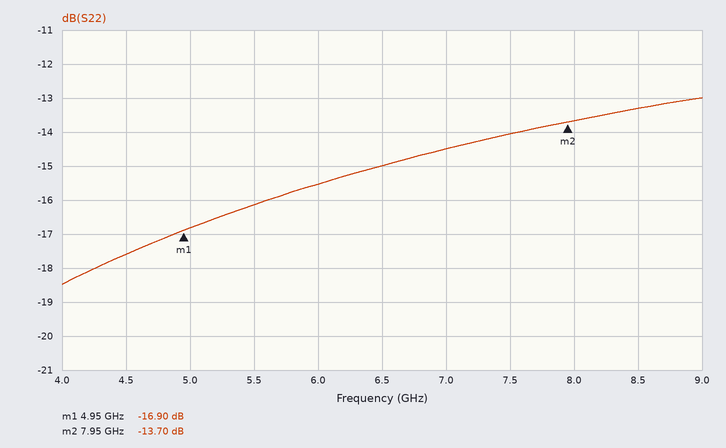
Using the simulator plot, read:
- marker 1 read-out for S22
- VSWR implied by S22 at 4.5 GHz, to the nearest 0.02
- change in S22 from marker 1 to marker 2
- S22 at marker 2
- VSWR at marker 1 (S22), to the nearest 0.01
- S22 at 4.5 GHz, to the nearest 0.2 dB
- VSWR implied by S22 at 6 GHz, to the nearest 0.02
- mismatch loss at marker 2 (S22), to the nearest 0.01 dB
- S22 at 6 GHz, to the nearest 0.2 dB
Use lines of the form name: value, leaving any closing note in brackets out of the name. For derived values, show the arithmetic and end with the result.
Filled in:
marker 1 read-out for S22: -16.90 dB
VSWR implied by S22 at 4.5 GHz, to the nearest 0.02: |Γ| = 10^(-17.6/20) = 0.1318; VSWR = (1 + 0.1318)/(1 − 0.1318) ≈ 1.30
change in S22 from marker 1 to marker 2: -13.7 − (-16.9) = 3.20 dB
S22 at marker 2: -13.70 dB
VSWR at marker 1 (S22), to the nearest 0.01: (1 + 0.1429)/(1 − 0.1429) ≈ 1.33
S22 at 4.5 GHz, to the nearest 0.2 dB: -17.6 dB
VSWR implied by S22 at 6 GHz, to the nearest 0.02: |Γ| = 10^(-15.6/20) = 0.1660; VSWR = (1 + 0.1660)/(1 − 0.1660) ≈ 1.40
mismatch loss at marker 2 (S22), to the nearest 0.01 dB: −10 log10(1 − 10^(-13.7/10)) ≈ 0.19 dB
S22 at 6 GHz, to the nearest 0.2 dB: -15.6 dB
